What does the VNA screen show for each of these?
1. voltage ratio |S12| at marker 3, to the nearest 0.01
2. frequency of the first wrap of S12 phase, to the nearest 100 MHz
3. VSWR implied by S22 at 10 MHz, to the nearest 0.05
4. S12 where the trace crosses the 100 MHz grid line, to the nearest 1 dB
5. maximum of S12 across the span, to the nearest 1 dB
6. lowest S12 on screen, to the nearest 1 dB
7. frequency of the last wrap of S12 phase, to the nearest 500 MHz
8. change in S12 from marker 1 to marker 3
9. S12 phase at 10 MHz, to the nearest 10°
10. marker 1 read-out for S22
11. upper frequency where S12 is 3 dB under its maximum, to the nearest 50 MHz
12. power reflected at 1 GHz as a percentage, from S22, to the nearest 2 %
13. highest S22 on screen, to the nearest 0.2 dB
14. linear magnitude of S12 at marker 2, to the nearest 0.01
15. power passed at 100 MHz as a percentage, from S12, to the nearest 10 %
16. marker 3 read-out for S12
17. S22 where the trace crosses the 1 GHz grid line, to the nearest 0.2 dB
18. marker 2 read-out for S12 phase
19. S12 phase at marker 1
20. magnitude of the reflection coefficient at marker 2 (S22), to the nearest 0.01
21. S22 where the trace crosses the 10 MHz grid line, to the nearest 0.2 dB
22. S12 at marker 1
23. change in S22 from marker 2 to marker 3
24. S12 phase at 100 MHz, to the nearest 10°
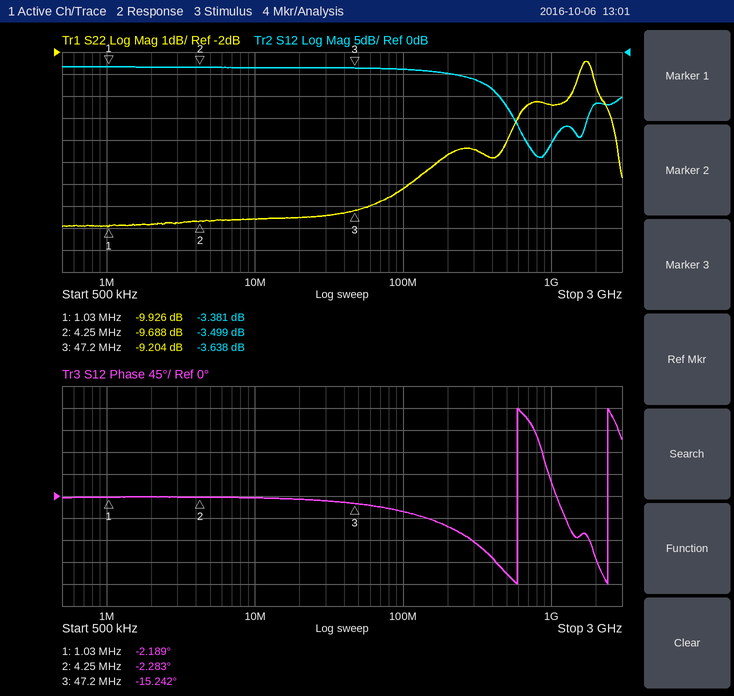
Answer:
0.66
600 MHz
2.00
-4 dB
-3 dB
-24 dB
2.5 GHz
-0.257 dB
0°
-9.926 dB
300 MHz
36 %
-2.4 dB
0.67
40 %
-3.638 dB
-4.4 dB
-2.283°
-2.189°
0.33
-9.6 dB
-3.381 dB
0.484 dB
-30°
